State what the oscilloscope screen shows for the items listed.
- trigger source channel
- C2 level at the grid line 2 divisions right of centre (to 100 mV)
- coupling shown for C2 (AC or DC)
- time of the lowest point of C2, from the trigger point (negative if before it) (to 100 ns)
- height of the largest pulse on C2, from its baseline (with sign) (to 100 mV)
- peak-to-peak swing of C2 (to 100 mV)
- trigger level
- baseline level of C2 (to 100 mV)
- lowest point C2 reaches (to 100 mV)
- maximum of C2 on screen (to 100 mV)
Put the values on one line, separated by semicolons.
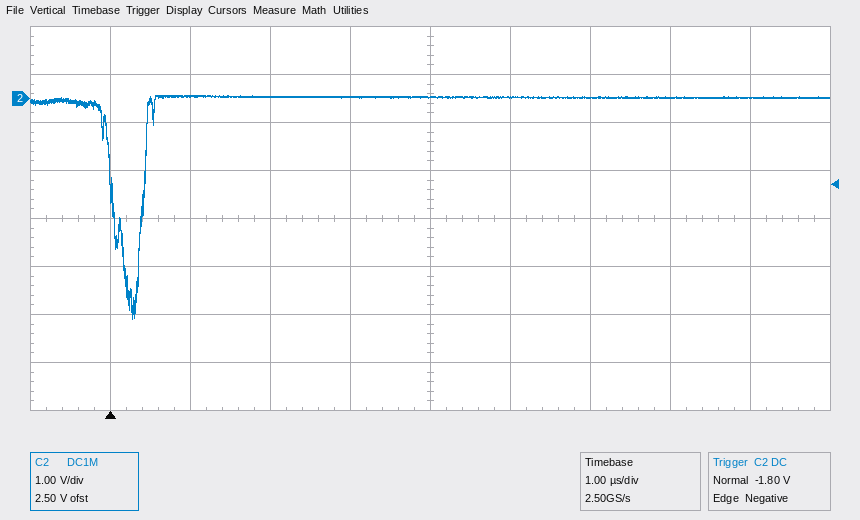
C2; 0.0 V; DC; +300 ns; -4.6 V; 4.7 V; -1.80 V; 0.0 V; -4.6 V; 100 mV
